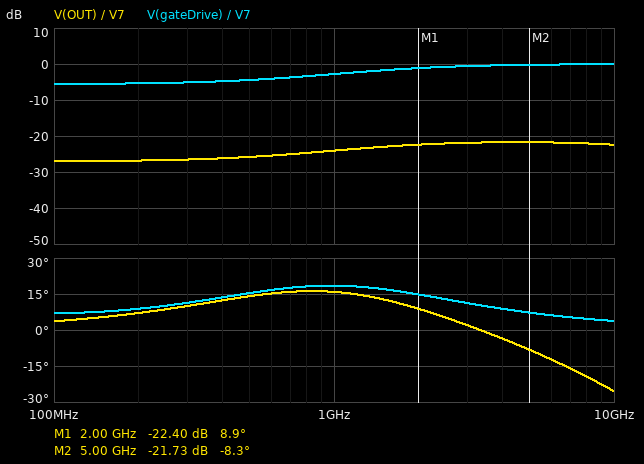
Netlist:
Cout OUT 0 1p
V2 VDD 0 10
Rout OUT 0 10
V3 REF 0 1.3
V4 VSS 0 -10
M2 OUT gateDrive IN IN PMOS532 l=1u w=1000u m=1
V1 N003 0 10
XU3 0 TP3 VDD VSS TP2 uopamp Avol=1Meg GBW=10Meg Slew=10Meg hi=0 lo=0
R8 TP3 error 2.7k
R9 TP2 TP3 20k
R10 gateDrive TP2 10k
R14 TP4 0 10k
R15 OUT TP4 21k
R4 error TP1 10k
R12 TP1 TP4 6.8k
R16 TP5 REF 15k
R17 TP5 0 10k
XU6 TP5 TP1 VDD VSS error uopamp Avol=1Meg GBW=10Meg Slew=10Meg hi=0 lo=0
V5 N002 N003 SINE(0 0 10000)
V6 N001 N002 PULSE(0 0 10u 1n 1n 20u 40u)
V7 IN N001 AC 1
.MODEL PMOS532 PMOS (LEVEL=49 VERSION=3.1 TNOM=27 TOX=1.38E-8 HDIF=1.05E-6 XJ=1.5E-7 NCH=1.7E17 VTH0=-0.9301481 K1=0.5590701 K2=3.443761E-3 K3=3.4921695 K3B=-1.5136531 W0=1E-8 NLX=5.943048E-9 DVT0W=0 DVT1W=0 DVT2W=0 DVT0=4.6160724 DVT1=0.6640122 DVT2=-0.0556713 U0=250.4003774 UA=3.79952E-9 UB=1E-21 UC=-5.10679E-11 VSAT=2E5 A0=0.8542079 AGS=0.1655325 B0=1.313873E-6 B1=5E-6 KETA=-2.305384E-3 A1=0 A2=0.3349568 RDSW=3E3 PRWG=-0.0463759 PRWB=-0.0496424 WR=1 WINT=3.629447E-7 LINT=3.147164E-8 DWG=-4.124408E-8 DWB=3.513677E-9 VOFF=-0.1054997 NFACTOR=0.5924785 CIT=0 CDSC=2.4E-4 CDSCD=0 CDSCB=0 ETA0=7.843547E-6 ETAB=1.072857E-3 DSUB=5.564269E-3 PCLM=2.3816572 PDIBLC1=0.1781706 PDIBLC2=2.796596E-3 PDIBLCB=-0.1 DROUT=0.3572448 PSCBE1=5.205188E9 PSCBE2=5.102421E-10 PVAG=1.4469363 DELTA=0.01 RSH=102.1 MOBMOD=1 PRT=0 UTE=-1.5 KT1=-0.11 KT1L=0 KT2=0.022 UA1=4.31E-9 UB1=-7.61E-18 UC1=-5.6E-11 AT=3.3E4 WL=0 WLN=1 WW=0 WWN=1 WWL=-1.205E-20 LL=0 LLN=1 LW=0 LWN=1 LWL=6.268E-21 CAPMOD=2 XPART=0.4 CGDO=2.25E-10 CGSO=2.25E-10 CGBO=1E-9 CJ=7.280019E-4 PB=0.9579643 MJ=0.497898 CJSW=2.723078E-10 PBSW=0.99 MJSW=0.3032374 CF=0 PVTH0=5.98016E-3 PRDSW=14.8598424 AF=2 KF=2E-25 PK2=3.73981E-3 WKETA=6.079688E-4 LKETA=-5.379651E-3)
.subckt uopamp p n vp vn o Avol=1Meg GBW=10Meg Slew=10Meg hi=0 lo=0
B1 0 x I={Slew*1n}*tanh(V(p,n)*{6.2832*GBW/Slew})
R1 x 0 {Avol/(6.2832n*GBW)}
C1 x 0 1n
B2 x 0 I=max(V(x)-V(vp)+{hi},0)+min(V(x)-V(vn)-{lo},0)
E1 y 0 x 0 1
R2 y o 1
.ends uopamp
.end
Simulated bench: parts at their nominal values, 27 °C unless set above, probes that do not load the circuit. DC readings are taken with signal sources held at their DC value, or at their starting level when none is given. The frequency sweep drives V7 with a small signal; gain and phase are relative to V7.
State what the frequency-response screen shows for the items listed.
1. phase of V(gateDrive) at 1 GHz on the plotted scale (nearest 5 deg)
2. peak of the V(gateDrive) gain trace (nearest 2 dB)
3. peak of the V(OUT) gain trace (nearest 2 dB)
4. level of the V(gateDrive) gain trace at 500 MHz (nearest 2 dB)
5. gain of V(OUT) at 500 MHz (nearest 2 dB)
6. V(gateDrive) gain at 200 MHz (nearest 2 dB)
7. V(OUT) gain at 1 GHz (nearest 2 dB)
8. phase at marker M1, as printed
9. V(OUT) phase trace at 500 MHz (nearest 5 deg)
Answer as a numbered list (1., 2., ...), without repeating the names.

1. 20 deg
2. 0 dB
3. -22 dB
4. -4 dB
5. -26 dB
6. -6 dB
7. -24 dB
8. 8.9 deg
9. 15 deg
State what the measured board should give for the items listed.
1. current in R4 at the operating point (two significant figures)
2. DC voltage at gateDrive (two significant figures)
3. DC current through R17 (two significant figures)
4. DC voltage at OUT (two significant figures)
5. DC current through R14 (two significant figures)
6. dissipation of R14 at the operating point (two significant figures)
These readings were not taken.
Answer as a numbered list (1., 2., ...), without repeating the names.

1. 28 µA
2. -5.9 V
3. 52 µA
4. 450 mV
5. 33 µA
6. 11 µW
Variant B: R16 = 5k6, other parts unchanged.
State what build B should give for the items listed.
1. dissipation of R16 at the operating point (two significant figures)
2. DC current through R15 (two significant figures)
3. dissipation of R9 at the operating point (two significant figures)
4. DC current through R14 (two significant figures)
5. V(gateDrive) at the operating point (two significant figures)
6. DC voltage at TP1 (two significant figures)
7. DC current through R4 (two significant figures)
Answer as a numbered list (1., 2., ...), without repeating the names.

1. 39 µW
2. 1.8 µA
3. 4.9 mW
4. 49 µA
5. -9.9 V
6. 830 mV
7. 51 µA
